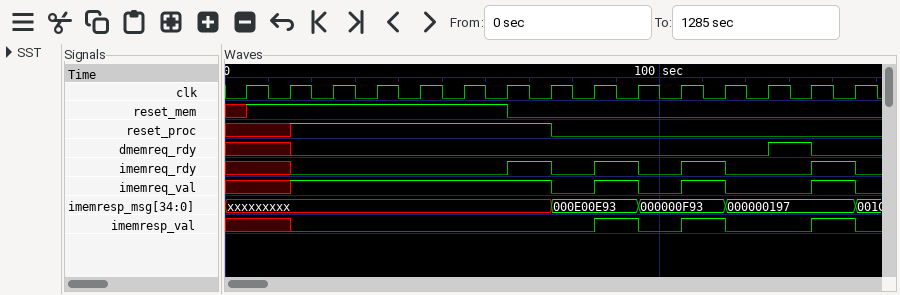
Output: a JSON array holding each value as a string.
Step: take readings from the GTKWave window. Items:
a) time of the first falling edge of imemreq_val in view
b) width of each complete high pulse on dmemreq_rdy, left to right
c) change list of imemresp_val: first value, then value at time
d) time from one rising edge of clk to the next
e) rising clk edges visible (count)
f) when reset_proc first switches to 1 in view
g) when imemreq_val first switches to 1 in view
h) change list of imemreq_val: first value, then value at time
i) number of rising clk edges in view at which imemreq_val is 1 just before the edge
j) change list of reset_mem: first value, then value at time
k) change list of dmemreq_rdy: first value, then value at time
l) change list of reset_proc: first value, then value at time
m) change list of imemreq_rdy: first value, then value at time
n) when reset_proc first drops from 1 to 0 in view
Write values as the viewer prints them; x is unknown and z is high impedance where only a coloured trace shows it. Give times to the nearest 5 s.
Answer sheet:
["75 s", "10 s", "x, 0 at 15 s, 1 at 85 s, 0 at 95 s, 1 at 105 s, 0 at 115 s, 1 at 135 s, 0 at 145 s", "10 s", "15", "15 s", "15 s", "x, 1 at 15 s, 0 at 75 s, 1 at 85 s, 0 at 95 s, 1 at 105 s, 0 at 115 s, 1 at 135 s, 0 at 145 s", "9", "x, 1 at 5 s, 0 at 65 s", "x, 0 at 15 s, 1 at 125 s, 0 at 135 s", "x, 1 at 15 s, 0 at 75 s", "x, 0 at 15 s, 1 at 65 s, 0 at 75 s, 1 at 85 s, 0 at 95 s, 1 at 105 s, 0 at 115 s, 1 at 135 s, 0 at 145 s", "75 s"]
